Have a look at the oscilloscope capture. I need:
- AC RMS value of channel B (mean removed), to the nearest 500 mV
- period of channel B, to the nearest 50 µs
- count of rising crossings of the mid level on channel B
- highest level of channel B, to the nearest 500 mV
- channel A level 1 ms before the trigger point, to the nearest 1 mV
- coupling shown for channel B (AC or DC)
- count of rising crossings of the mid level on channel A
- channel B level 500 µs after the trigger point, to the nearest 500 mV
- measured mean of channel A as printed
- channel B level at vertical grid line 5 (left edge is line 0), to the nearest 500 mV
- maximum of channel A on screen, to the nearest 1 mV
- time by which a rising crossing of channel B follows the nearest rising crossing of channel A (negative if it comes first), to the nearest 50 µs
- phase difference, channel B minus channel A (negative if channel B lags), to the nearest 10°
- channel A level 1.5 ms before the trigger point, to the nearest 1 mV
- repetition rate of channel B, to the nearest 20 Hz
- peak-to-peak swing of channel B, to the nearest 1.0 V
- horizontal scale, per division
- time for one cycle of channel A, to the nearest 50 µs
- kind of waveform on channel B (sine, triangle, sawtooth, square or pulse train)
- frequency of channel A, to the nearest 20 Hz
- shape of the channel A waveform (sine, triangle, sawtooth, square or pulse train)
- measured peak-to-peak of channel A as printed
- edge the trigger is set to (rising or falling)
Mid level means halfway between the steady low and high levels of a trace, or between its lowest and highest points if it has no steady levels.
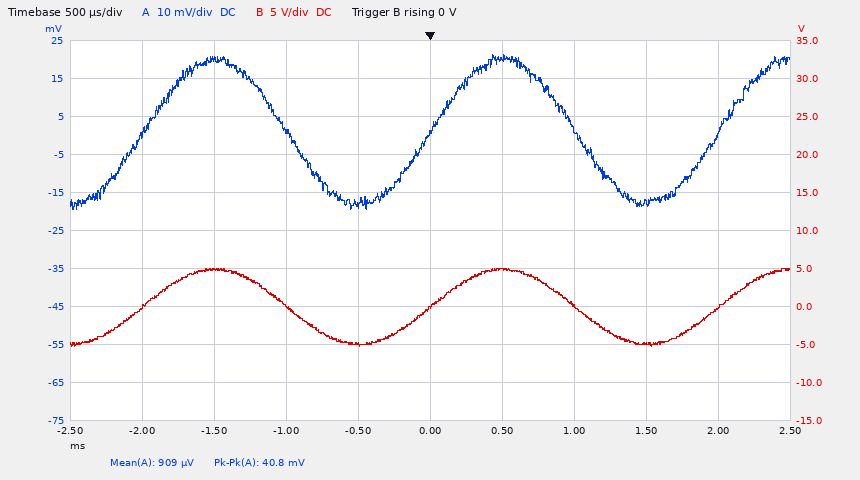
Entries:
3.5 V
2.00 ms
3
5.0 V
1 mV
DC
3
5.0 V
909 µV
0.0 V
21 mV
0 µs
0°
20 mV
500 Hz
10.0 V
500 µs
2.00 ms
sine
500 Hz
sine
40.8 mV
rising
